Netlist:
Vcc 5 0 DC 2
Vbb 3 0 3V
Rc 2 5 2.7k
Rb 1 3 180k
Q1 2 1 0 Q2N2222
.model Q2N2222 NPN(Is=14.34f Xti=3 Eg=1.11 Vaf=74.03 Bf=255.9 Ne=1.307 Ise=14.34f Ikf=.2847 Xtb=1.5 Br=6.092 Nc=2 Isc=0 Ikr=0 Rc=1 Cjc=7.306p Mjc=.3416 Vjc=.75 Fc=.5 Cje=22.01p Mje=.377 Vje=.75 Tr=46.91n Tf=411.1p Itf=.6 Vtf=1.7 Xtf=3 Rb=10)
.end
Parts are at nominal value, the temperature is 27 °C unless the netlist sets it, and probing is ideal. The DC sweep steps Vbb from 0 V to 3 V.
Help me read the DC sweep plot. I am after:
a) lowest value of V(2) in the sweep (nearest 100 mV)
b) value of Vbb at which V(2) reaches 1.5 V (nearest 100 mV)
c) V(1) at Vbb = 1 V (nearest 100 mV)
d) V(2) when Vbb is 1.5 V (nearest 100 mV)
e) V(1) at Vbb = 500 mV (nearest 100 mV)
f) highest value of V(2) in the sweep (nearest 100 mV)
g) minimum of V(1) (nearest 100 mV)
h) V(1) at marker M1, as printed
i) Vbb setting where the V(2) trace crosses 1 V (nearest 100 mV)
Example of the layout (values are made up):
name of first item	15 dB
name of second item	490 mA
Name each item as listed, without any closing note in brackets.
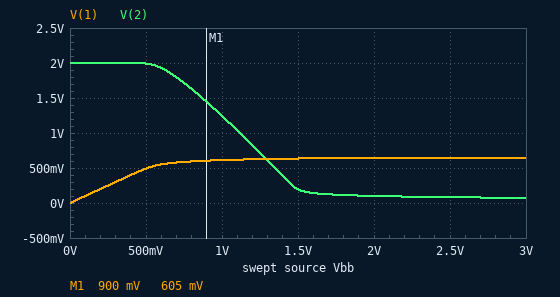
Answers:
lowest value of V(2) in the sweep	100 mV
value of Vbb at which V(2) reaches 1.5 V	900 mV
V(1) at Vbb = 1 V	600 mV
V(2) when Vbb is 1.5 V	200 mV
V(1) at Vbb = 500 mV	500 mV
highest value of V(2) in the sweep	2.0 V
minimum of V(1)	0 V
V(1) at marker M1, as printed	605 mV
Vbb setting where the V(2) trace crosses 1 V	1.1 V
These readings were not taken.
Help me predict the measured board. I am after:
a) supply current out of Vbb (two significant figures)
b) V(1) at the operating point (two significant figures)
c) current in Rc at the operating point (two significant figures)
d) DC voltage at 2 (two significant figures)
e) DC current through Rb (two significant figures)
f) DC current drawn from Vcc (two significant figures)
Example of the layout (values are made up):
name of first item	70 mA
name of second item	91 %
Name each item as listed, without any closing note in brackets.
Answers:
supply current out of Vbb	13 µA
V(1) at the operating point	640 mV
current in Rc at the operating point	710 µA
DC voltage at 2	73 mV
DC current through Rb	13 µA
DC current drawn from Vcc	710 µA
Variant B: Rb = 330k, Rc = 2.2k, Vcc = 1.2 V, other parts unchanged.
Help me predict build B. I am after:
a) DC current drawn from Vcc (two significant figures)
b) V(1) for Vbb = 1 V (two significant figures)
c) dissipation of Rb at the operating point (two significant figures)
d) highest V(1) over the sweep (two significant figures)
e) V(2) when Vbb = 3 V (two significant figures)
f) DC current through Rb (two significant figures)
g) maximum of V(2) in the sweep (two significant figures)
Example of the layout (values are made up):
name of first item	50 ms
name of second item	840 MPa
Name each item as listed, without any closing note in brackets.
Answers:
DC current drawn from Vcc	510 µA
V(1) for Vbb = 1 V	600 mV
dissipation of Rb at the operating point	17 µW
highest V(1) over the sweep	630 mV
V(2) when Vbb = 3 V	85 mV
DC current through Rb	7.2 µA
maximum of V(2) in the sweep	1.2 V
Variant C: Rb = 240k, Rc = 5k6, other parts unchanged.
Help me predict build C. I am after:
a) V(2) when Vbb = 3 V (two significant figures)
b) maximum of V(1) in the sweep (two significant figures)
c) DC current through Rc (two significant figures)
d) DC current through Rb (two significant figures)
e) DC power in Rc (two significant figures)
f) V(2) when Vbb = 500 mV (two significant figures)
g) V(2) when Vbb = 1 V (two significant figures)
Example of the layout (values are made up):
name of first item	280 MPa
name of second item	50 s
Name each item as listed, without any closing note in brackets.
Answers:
V(2) when Vbb = 3 V	58 mV
maximum of V(1) in the sweep	620 mV
DC current through Rc	350 µA
DC current through Rb	9.9 µA
DC power in Rc	670 µW
V(2) when Vbb = 500 mV	2.0 V
V(2) when Vbb = 1 V	850 mV
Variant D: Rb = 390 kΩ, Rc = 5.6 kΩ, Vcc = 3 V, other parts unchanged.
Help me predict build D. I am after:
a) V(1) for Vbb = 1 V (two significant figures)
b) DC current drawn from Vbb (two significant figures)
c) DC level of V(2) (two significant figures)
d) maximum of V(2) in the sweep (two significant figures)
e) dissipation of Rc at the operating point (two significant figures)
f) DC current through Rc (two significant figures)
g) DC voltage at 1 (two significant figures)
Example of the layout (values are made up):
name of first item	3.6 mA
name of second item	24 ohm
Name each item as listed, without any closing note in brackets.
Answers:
V(1) for Vbb = 1 V	590 mV
DC current drawn from Vbb	6.1 µA
DC level of V(2)	96 mV
maximum of V(2) in the sweep	3.0 V
dissipation of Rc at the operating point	1.5 mW
DC current through Rc	520 µA
DC voltage at 1	630 mV
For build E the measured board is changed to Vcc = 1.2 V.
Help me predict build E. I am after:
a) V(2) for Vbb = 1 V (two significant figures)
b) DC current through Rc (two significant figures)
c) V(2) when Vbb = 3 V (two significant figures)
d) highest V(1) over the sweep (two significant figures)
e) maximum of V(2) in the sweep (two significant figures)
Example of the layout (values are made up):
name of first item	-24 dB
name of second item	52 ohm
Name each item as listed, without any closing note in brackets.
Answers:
V(2) for Vbb = 1 V	450 mV
DC current through Rc	420 µA
V(2) when Vbb = 3 V	56 mV
highest V(1) over the sweep	630 mV
maximum of V(2) in the sweep	1.2 V
